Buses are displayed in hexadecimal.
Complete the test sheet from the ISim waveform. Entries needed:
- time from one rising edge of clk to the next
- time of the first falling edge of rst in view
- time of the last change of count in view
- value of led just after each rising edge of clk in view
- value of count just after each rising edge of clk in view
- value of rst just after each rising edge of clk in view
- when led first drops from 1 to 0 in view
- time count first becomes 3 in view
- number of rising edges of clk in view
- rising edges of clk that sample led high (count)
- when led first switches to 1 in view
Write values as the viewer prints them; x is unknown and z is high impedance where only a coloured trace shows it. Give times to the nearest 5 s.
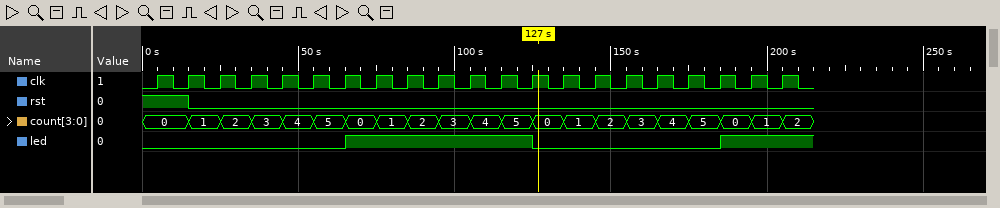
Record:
10 s
15 s
205 s
0 0 0 0 0 0 1 1 1 1 1 1 0 0 0 0 0 0 1 1 1
0, 1, 2, 3, 4, 5, 0, 1, 2, 3, 4, 5, 0, 1, 2, 3, 4, 5, 0, 1, 2
1 0 0 0 0 0 0 0 0 0 0 0 0 0 0 0 0 0 0 0 0
125 s
35 s
21
8
65 s
